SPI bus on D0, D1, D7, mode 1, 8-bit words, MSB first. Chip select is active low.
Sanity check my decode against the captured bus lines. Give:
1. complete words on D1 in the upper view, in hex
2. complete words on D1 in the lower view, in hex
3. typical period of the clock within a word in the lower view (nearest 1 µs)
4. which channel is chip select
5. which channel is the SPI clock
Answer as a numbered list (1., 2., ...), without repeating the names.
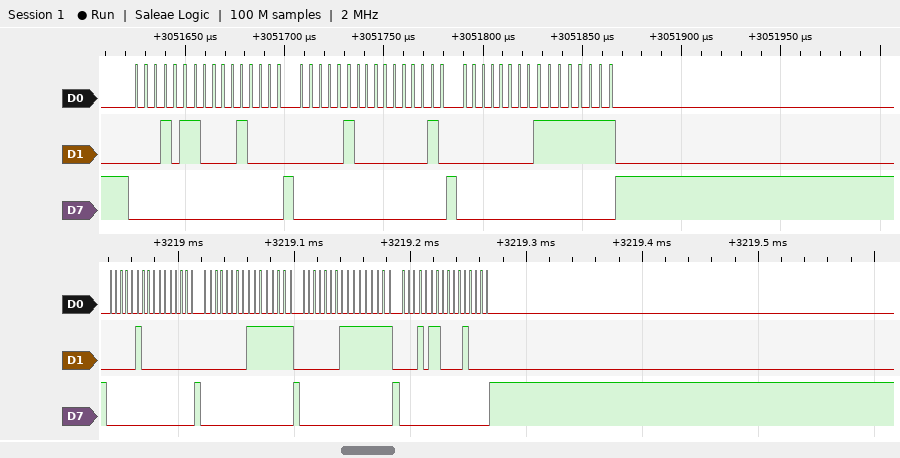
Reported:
1. 16, 10, 04, 02, 00, FF
2. 04, 00, 00, FF, 01, FF, 16, 10
3. 5 µs
4. D7
5. D0
